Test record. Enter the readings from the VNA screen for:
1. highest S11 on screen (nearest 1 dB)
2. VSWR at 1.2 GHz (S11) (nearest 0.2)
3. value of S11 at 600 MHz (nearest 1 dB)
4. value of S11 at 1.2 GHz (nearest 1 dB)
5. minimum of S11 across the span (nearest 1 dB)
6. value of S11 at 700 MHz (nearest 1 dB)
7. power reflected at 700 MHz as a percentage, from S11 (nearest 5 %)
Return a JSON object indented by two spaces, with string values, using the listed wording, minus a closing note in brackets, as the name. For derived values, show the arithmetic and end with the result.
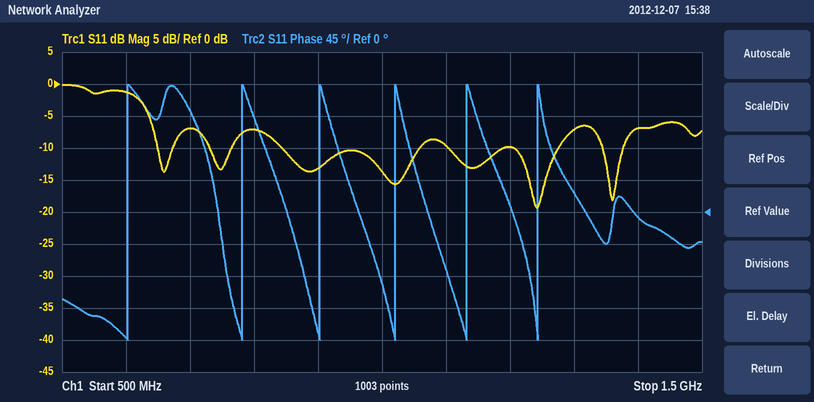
{
  "highest S11 on screen": "0 dB",
  "VSWR at 1.2 GHz (S11)": "|Γ| = 10^(-10/20) = 0.3162; VSWR = (1 + 0.3162)/(1 − 0.3162) ≈ 1.92, so 2.0 to the nearest 0.2",
  "value of S11 at 600 MHz": "-1 dB",
  "value of S11 at 1.2 GHz": "-10 dB",
  "minimum of S11 across the span": "-19 dB",
  "value of S11 at 700 MHz": "-7 dB",
  "power reflected at 700 MHz as a percentage, from S11": "10^(-7/10) ≈ 20 %"
}
